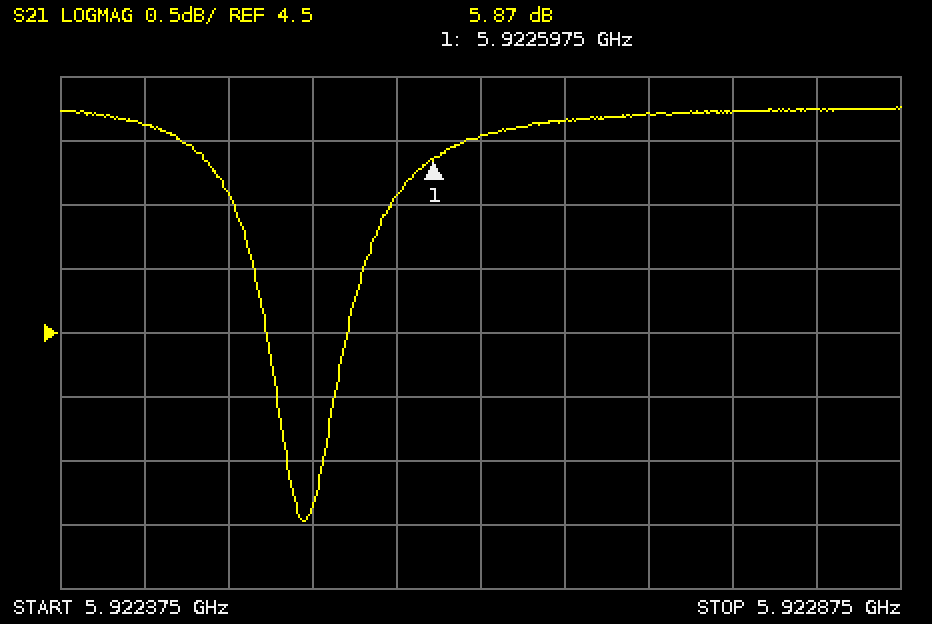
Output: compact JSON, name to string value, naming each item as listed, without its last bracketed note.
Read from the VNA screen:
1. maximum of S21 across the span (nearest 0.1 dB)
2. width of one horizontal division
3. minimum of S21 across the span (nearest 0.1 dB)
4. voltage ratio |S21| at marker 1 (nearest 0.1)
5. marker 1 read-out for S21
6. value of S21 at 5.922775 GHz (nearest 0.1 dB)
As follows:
{"maximum of S21 across the span": "6.3 dB", "width of one horizontal division": "50 kHz", "minimum of S21 across the span": "3.0 dB", "voltage ratio |S21| at marker 1": "2.0", "marker 1 read-out for S21": "5.87 dB", "value of S21 at 5.922775 GHz": "6.2 dB"}
